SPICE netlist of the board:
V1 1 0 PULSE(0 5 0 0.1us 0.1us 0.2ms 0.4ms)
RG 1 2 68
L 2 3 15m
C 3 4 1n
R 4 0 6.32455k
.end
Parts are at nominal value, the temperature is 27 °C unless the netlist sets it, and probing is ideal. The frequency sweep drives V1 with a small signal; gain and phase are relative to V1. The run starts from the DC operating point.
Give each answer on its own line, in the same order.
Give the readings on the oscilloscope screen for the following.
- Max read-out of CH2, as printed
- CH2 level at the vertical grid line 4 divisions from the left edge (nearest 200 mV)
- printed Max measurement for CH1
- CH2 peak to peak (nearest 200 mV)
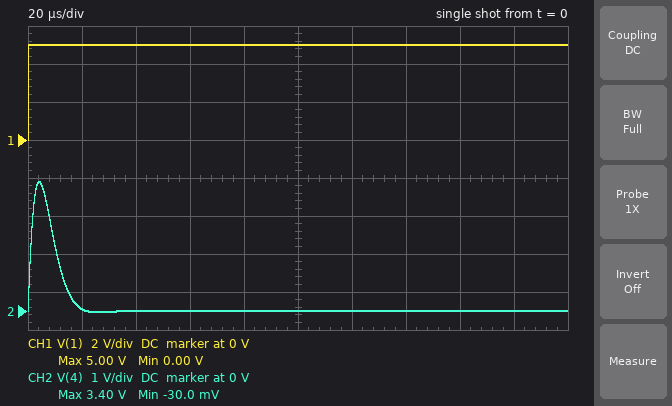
3.40 V
0 V
5.00 V
3.4 V
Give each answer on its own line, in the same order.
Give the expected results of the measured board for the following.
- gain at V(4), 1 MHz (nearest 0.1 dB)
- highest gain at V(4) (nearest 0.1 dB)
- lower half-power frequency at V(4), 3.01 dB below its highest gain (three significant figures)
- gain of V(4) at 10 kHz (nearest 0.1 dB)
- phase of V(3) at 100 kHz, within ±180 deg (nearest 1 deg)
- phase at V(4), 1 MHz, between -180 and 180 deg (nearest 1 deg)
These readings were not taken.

-23.5 dB
-0.1 dB
19.4 kHz
-8.2 dB
-65 deg
-86 deg
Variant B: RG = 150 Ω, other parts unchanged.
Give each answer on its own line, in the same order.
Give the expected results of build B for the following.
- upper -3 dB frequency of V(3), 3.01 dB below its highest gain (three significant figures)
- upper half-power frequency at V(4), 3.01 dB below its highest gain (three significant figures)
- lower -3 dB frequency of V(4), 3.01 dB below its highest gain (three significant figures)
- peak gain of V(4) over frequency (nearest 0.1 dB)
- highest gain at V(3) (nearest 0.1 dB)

72.3 kHz
87.9 kHz
19.2 kHz
-0.2 dB
1.5 dB
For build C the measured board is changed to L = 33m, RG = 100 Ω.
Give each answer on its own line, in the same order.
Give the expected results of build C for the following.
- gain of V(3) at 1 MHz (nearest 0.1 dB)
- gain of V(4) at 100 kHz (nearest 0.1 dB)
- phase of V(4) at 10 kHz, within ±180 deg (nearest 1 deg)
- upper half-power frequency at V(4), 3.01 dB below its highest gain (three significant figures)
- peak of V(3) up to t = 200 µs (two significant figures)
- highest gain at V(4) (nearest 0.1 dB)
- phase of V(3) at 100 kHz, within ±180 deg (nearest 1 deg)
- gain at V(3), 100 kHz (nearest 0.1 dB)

-30.3 dB
-10.1 dB
65 deg
47.2 kHz
6.3 V
-0.1 dB
-86 deg
-9.8 dB
